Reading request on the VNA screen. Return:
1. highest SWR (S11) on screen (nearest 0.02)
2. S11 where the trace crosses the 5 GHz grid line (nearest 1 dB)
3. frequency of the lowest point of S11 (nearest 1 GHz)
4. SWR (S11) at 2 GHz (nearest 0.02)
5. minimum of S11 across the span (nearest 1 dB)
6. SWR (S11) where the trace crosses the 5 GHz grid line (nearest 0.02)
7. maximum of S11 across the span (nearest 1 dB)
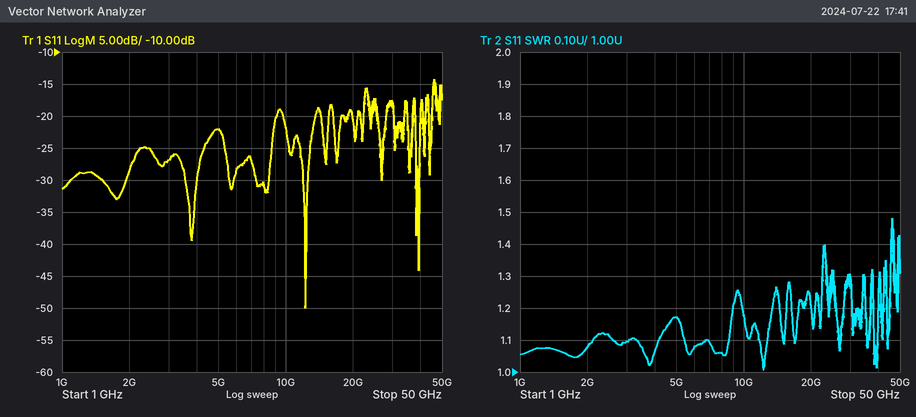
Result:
1.48
-22 dB
12 GHz
1.08
-50 dB
1.18
-14 dB
